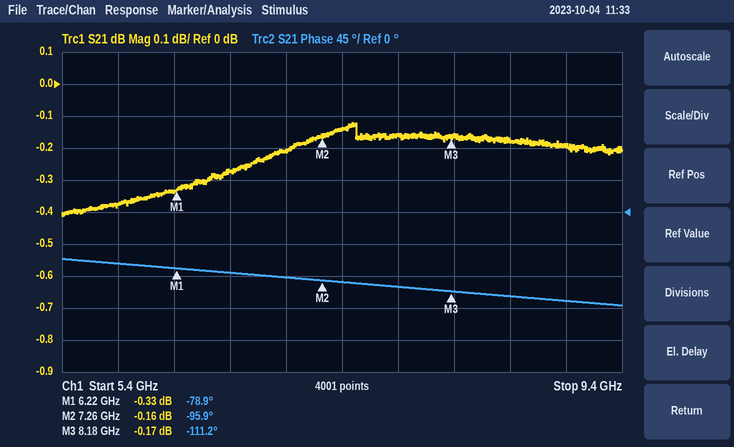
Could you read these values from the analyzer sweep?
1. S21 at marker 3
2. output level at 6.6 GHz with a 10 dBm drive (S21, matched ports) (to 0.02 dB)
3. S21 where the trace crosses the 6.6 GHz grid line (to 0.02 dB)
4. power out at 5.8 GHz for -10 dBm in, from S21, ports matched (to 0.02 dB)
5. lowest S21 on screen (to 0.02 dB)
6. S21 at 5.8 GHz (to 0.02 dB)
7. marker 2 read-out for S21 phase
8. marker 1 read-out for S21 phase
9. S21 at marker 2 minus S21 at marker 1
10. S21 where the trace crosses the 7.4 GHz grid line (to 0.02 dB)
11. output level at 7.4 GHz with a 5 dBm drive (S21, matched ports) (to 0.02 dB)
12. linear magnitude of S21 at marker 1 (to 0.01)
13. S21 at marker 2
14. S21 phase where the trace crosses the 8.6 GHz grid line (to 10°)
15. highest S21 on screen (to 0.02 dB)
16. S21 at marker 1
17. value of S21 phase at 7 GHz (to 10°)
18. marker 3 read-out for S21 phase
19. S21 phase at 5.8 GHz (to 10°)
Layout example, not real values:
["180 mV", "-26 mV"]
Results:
["-0.17 dB", "9.72 dBm", "-0.28 dB", "-10.38 dBm", "-0.42 dB", "-0.38 dB", "-95.9°", "-78.9°", "0.17 dB", "-0.14 dB", "4.86 dBm", "0.96", "-0.16 dB", "-120°", "-0.12 dB", "-0.33 dB", "-90°", "-111.2°", "-70°"]
